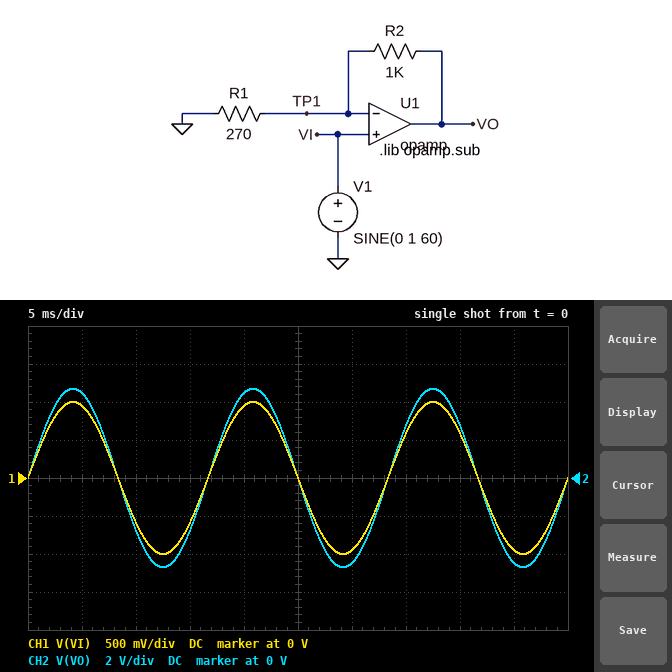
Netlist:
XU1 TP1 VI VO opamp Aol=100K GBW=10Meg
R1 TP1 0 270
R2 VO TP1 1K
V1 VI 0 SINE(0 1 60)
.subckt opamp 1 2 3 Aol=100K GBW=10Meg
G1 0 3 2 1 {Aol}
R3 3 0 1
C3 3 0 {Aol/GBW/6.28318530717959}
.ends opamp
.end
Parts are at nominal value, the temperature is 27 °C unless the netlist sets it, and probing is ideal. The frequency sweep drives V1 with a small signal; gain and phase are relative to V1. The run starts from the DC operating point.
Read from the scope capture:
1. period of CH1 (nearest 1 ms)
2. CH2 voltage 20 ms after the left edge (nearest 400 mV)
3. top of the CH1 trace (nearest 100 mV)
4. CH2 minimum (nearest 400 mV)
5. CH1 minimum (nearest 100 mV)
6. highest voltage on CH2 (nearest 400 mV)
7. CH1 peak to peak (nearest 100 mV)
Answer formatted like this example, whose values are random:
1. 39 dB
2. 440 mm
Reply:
1. 17 ms
2. 4.4 V
3. 1.0 V
4. -4.8 V
5. -1.0 V
6. 4.8 V
7. 2.0 V
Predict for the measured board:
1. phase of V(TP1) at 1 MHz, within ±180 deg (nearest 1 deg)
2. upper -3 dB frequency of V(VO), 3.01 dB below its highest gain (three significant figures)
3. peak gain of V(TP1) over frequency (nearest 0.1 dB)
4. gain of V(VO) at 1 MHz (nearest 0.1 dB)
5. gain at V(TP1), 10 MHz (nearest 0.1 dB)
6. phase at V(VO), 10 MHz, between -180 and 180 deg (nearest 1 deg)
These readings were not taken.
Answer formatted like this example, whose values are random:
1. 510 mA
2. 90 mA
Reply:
1. -25 deg
2. 2.13 MHz
3. 0 dB
4. 12.6 dB
5. -13.6 dB
6. -78 deg
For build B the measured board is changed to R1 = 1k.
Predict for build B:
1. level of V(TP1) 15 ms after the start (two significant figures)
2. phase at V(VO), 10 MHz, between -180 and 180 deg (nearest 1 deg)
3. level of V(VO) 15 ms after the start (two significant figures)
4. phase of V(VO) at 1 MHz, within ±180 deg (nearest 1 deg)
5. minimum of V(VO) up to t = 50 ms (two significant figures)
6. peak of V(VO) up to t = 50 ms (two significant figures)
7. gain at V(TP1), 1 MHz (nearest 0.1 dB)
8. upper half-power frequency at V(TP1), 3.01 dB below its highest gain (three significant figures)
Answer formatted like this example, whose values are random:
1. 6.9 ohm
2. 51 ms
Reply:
1. -590 mV
2. -63 deg
3. -1.2 V
4. -11 deg
5. -2.0 V
6. 2.0 V
7. -0.2 dB
8. 5.00 MHz
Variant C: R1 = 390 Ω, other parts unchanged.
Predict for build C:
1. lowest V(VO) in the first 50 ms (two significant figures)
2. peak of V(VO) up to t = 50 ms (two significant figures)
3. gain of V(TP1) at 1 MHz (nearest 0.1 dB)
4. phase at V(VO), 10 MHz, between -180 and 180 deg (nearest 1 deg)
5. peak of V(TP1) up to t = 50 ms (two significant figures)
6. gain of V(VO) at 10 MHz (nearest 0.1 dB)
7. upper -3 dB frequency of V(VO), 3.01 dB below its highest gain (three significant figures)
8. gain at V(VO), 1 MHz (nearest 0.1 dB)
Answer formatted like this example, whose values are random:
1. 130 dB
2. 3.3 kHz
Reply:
1. -3.6 V
2. 3.6 V
3. -0.5 dB
4. -74 deg
5. 1.0 V
6. -0.3 dB
7. 2.81 MHz
8. 10.5 dB
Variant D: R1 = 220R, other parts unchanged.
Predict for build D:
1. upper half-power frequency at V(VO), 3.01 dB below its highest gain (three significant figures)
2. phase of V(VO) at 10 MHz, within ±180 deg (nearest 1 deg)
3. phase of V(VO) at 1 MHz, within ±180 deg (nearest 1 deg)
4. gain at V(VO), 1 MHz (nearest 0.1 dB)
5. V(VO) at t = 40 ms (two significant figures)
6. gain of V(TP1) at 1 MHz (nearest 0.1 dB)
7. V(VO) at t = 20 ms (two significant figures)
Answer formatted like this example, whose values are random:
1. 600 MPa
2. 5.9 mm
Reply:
1. 1.80 MHz
2. -80 deg
3. -29 deg
4. 13.7 dB
5. 3.3 V
6. -1.2 dB
7. 5.3 V
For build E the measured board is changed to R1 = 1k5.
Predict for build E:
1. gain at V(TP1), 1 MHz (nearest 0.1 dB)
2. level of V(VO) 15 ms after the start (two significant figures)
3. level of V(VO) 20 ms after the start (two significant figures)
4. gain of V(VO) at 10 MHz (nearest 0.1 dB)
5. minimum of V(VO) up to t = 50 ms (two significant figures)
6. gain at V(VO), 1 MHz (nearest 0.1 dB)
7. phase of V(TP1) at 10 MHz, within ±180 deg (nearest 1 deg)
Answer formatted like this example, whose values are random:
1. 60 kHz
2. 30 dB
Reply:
1. -0.1 dB
2. -980 mV
3. 1.6 V
4. -1.3 dB
5. -1.7 V
6. 4.3 dB
7. -59 deg
